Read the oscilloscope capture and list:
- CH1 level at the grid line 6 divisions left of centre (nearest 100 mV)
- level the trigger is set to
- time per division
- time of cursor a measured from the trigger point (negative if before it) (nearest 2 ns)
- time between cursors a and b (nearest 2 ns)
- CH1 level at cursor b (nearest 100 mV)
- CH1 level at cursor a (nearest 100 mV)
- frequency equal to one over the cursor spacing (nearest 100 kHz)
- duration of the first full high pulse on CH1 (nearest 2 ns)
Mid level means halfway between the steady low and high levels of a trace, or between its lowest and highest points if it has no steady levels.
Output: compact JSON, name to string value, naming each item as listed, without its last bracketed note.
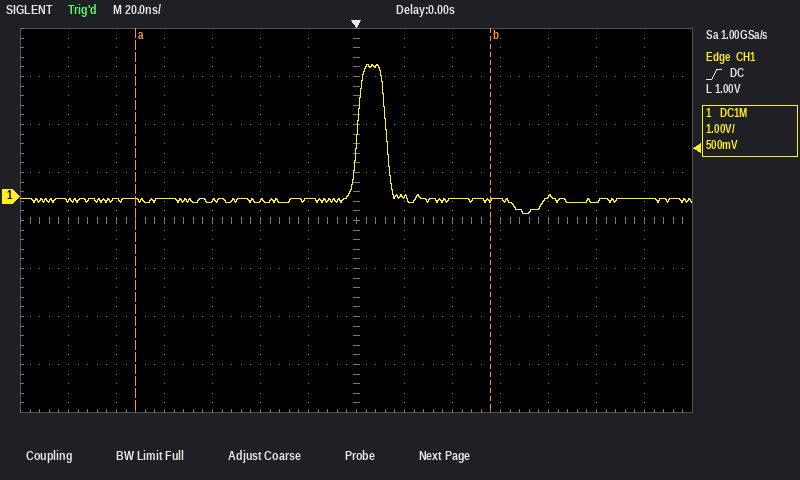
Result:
{"CH1 level at the grid line 6 divisions left of centre": "-100 mV", "level the trigger is set to": "1.00 V", "time per division": "20 ns", "time of cursor a measured from the trigger point (negative if before it)": "-92 ns", "time between cursors a and b": "148 ns", "CH1 level at cursor b": "-100 mV", "CH1 level at cursor a": "-100 mV", "frequency equal to one over the cursor spacing": "6.8 MHz", "duration of the first full high pulse on CH1": "12 ns"}
